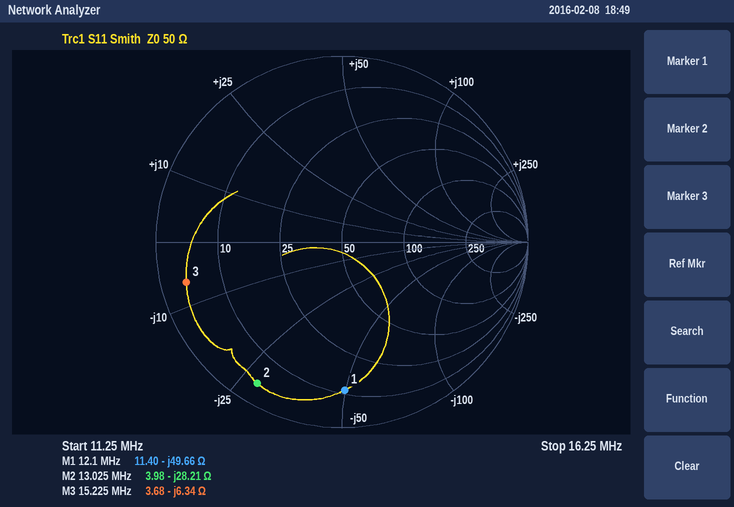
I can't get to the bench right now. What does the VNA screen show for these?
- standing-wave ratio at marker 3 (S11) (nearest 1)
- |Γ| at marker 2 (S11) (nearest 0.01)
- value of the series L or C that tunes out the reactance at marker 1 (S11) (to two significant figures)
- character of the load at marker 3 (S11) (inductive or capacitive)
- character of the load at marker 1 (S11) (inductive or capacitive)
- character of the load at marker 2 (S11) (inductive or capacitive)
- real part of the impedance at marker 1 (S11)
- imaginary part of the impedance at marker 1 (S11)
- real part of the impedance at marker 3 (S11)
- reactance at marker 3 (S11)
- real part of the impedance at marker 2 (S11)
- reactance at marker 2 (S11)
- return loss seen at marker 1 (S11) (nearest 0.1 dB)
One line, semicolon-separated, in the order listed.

14; 0.89; 650 nH; capacitive; capacitive; capacitive; 11.40 Ω; -49.66 Ω; 3.68 Ω; -6.34 Ω; 3.98 Ω; -28.21 Ω; 2.0 dB
